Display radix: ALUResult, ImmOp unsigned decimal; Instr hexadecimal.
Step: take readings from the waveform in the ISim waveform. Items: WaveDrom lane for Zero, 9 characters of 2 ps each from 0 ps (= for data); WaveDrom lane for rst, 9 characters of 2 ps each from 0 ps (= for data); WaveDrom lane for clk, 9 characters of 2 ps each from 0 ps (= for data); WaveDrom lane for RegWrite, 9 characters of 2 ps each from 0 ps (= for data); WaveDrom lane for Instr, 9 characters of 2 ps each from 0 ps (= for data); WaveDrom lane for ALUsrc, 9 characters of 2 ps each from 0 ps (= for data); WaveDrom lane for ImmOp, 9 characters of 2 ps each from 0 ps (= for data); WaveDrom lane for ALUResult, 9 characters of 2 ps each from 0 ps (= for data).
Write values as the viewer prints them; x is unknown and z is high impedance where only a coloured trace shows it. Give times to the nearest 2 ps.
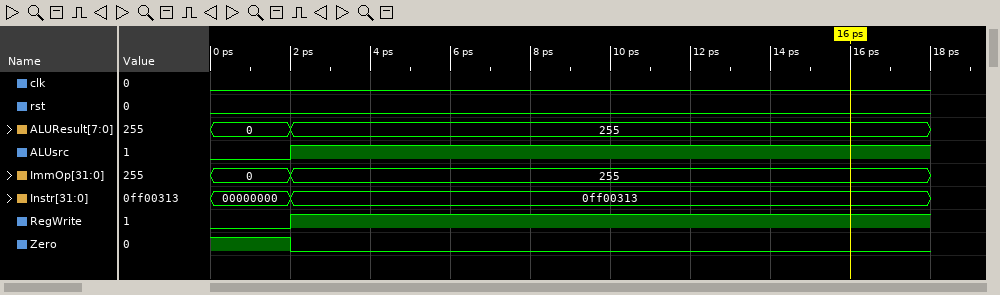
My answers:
{name: 'Zero', wave: '10.......'}
{name: 'rst', wave: '0........'}
{name: 'clk', wave: '0........'}
{name: 'RegWrite', wave: '01.......'}
{name: 'Instr', wave: '==.......', data: '00000000 0ff00313'}
{name: 'ALUsrc', wave: '01.......'}
{name: 'ImmOp', wave: '==.......', data: '0 255'}
{name: 'ALUResult', wave: '==.......', data: '0 255'}
